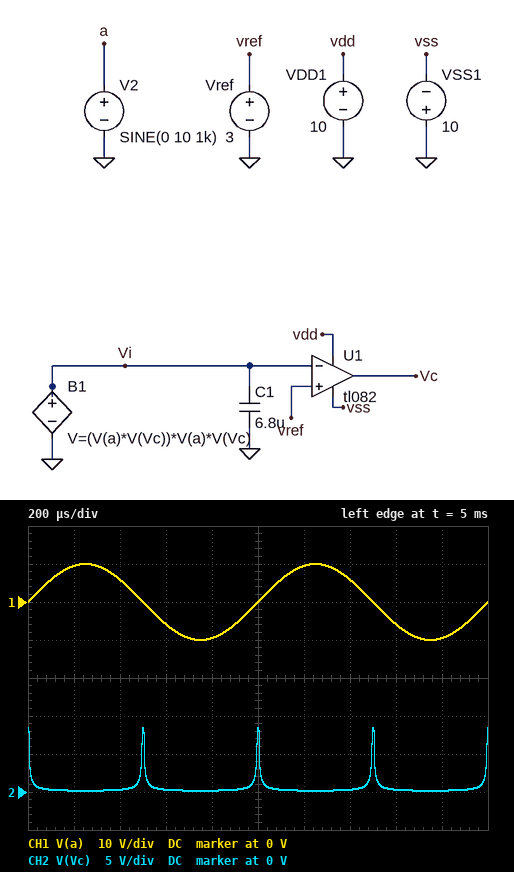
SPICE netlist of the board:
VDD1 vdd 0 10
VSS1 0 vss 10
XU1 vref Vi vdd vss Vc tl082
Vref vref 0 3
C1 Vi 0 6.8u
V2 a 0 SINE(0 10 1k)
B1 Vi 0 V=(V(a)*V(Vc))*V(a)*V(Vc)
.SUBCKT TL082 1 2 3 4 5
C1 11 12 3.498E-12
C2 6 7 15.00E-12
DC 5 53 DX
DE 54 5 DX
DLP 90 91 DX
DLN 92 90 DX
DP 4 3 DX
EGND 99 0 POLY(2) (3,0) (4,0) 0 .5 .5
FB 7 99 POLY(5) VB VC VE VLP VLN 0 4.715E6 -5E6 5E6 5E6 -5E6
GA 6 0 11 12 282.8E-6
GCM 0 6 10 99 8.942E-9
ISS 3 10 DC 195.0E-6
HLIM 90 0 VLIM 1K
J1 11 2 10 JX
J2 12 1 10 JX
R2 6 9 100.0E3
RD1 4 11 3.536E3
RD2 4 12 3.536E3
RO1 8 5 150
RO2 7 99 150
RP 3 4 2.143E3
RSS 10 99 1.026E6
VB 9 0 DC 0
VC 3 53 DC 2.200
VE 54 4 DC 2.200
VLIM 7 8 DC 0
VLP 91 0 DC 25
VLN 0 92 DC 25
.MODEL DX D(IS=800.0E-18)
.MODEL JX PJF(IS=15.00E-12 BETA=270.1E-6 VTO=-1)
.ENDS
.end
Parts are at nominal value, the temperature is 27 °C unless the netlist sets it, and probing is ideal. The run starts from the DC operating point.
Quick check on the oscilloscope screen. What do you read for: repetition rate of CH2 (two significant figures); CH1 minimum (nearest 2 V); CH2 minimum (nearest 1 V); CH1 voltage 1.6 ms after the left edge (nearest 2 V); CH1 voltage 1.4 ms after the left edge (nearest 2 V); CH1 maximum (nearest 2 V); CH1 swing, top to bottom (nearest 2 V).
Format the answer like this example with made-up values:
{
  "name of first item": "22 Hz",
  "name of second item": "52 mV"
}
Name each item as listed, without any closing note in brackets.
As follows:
{
  "repetition rate of CH2": "2.0 kHz",
  "CH1 minimum": "-10 V",
  "CH2 minimum": "0 V",
  "CH1 voltage 1.6 ms after the left edge": "-6 V",
  "CH1 voltage 1.4 ms after the left edge": "6 V",
  "CH1 maximum": "10 V",
  "CH1 swing, top to bottom": "20 V"
}
